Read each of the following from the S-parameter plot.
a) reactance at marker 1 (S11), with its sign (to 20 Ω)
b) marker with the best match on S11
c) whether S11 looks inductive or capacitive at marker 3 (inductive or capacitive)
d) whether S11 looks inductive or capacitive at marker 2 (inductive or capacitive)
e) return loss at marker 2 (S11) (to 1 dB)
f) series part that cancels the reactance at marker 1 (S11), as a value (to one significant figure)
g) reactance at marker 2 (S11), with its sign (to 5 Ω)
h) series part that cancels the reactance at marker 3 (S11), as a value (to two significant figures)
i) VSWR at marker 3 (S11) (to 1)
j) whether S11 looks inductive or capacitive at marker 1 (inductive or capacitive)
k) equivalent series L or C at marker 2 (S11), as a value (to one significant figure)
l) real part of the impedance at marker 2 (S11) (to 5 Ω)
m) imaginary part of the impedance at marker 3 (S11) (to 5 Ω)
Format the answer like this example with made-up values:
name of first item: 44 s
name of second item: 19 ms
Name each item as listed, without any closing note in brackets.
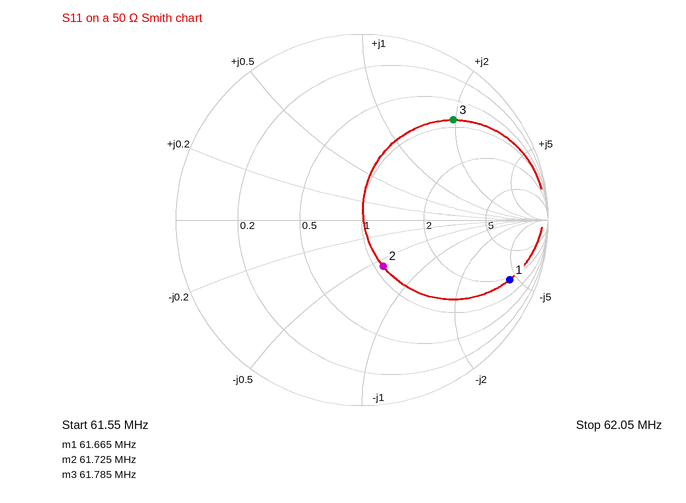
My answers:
reactance at marker 1 (S11), with its sign: -220 Ω
marker with the best match on S11: marker 2
whether S11 looks inductive or capacitive at marker 3: inductive
whether S11 looks inductive or capacitive at marker 2: capacitive
return loss at marker 2 (S11): 11 dB
series part that cancels the reactance at marker 1 (S11), as a value: 600 nH
reactance at marker 2 (S11), with its sign: -30 Ω
series part that cancels the reactance at marker 3 (S11), as a value: 26 pF
VSWR at marker 3 (S11): 6
whether S11 looks inductive or capacitive at marker 1: capacitive
equivalent series L or C at marker 2 (S11), as a value: 90 pF
real part of the impedance at marker 2 (S11): 55 Ω
imaginary part of the impedance at marker 3 (S11): +100 Ω
